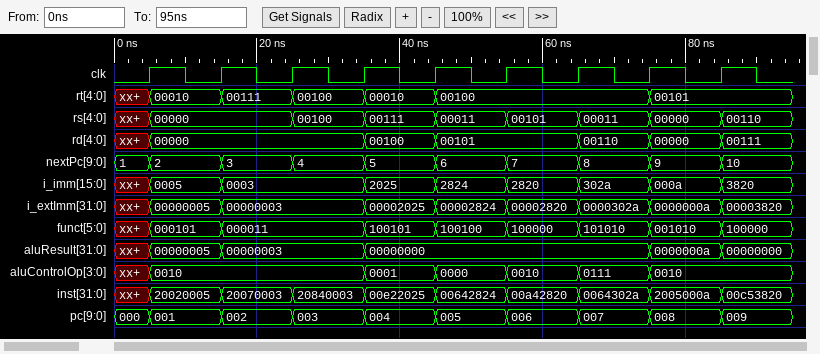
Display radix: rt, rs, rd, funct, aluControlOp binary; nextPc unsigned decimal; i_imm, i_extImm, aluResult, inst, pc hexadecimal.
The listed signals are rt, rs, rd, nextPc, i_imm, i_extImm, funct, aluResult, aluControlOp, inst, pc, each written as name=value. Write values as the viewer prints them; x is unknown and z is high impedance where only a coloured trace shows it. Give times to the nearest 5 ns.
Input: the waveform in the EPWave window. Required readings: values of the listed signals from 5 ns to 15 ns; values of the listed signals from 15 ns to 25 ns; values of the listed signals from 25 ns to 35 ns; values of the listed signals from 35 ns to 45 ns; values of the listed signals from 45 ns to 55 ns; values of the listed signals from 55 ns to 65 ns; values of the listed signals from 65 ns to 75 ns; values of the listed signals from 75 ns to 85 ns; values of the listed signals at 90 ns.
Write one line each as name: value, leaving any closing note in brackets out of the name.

values of the listed signals from 5 ns to 15 ns: rt=00010, rs=00000, rd=00000, nextPc=2, i_imm=0005, i_extImm=00000005, funct=000101, aluResult=00000005, aluControlOp=0010, inst=20020005, pc=001
values of the listed signals from 15 ns to 25 ns: rt=00111, rs=00000, rd=00000, nextPc=3, i_imm=0003, i_extImm=00000003, funct=000011, aluResult=00000003, aluControlOp=0010, inst=20070003, pc=002
values of the listed signals from 25 ns to 35 ns: rt=00100, rs=00100, rd=00000, nextPc=4, i_imm=0003, i_extImm=00000003, funct=000011, aluResult=00000003, aluControlOp=0010, inst=20840003, pc=003
values of the listed signals from 35 ns to 45 ns: rt=00010, rs=00111, rd=00100, nextPc=5, i_imm=2025, i_extImm=00002025, funct=100101, aluResult=00000000, aluControlOp=0001, inst=00e22025, pc=004
values of the listed signals from 45 ns to 55 ns: rt=00100, rs=00011, rd=00101, nextPc=6, i_imm=2824, i_extImm=00002824, funct=100100, aluResult=00000000, aluControlOp=0000, inst=00642824, pc=005
values of the listed signals from 55 ns to 65 ns: rt=00100, rs=00101, rd=00101, nextPc=7, i_imm=2820, i_extImm=00002820, funct=100000, aluResult=00000000, aluControlOp=0010, inst=00a42820, pc=006
values of the listed signals from 65 ns to 75 ns: rt=00100, rs=00011, rd=00110, nextPc=8, i_imm=302a, i_extImm=0000302a, funct=101010, aluResult=00000000, aluControlOp=0111, inst=0064302a, pc=007
values of the listed signals from 75 ns to 85 ns: rt=00101, rs=00000, rd=00000, nextPc=9, i_imm=000a, i_extImm=0000000a, funct=001010, aluResult=0000000a, aluControlOp=0010, inst=2005000a, pc=008
values of the listed signals at 90 ns: rt=00101, rs=00110, rd=00111, nextPc=10, i_imm=3820, i_extImm=00003820, funct=100000, aluResult=00000000, aluControlOp=0010, inst=00c53820, pc=009
